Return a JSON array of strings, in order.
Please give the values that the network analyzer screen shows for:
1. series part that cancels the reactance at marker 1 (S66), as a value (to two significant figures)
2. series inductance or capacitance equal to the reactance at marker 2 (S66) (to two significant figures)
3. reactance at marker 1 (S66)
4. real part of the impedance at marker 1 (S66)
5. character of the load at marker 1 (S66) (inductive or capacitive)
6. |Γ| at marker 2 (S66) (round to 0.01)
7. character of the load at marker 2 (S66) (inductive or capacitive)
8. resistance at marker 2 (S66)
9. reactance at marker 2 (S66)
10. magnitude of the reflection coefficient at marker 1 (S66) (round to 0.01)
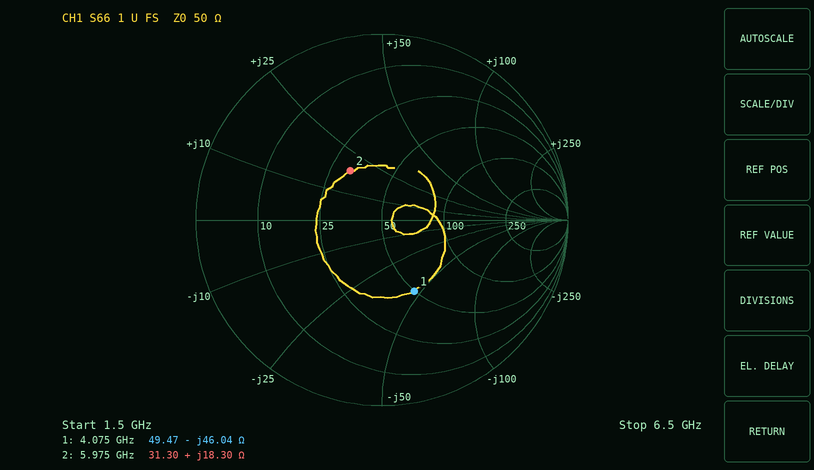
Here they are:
["1.8 nH", "490 pH", "-46.04 Ω", "49.47 Ω", "capacitive", "0.31", "inductive", "31.30 Ω", "+18.30 Ω", "0.42"]
